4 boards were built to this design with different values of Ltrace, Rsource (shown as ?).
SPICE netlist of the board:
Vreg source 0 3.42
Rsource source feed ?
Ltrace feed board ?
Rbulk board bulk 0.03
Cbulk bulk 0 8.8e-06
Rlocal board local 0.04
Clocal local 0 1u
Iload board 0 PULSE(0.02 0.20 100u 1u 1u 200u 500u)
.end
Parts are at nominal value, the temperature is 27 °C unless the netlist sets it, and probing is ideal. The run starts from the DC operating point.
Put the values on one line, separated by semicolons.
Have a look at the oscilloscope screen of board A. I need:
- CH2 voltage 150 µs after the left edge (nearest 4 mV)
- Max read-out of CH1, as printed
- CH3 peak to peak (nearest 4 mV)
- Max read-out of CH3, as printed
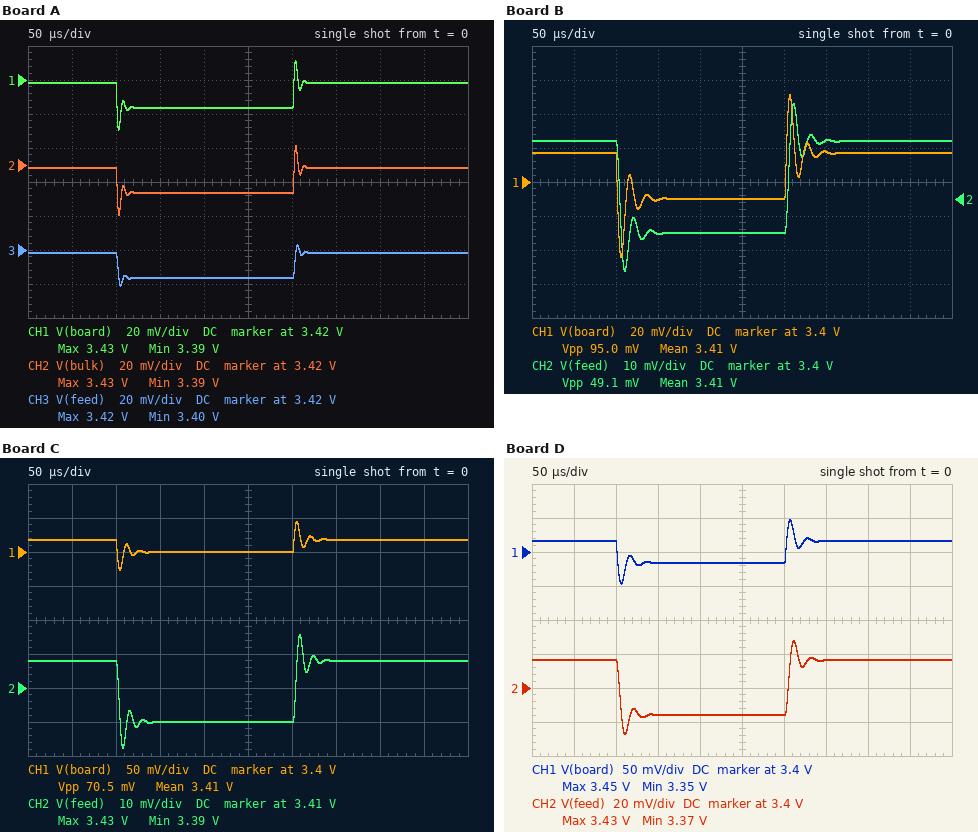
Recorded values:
3.404 V; 3.43 V; 24 mV; 3.42 V
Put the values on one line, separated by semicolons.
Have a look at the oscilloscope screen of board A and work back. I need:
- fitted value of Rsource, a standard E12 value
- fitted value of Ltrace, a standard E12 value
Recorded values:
0.082 Ω; 220 nH
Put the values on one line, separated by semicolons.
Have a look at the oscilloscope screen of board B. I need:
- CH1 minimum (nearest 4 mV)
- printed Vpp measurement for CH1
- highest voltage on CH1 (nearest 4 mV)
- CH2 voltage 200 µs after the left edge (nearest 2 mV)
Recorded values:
3.356 V; 95.0 mV; 3.452 V; 3.390 V
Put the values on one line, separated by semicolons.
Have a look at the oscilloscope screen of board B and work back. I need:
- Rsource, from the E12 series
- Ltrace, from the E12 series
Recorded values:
0.15 Ω; 1 µH
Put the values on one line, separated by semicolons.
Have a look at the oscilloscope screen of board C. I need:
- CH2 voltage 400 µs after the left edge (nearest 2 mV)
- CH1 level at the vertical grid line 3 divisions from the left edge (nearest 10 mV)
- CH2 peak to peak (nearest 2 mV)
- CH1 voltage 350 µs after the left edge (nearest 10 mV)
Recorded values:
3.418 V; 3.40 V; 34 mV; 3.42 V
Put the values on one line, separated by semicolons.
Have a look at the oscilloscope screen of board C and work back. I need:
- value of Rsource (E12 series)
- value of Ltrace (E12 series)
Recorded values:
0.1 Ω; 560 nH
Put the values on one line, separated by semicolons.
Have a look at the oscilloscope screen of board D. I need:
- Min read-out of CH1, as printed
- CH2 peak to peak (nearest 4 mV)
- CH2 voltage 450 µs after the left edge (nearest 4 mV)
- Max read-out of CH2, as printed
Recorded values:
3.35 V; 56 mV; 3.416 V; 3.43 V
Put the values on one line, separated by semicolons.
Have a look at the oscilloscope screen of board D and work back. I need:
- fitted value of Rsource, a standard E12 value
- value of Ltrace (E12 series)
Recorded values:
0.18 Ω; 1 µH
